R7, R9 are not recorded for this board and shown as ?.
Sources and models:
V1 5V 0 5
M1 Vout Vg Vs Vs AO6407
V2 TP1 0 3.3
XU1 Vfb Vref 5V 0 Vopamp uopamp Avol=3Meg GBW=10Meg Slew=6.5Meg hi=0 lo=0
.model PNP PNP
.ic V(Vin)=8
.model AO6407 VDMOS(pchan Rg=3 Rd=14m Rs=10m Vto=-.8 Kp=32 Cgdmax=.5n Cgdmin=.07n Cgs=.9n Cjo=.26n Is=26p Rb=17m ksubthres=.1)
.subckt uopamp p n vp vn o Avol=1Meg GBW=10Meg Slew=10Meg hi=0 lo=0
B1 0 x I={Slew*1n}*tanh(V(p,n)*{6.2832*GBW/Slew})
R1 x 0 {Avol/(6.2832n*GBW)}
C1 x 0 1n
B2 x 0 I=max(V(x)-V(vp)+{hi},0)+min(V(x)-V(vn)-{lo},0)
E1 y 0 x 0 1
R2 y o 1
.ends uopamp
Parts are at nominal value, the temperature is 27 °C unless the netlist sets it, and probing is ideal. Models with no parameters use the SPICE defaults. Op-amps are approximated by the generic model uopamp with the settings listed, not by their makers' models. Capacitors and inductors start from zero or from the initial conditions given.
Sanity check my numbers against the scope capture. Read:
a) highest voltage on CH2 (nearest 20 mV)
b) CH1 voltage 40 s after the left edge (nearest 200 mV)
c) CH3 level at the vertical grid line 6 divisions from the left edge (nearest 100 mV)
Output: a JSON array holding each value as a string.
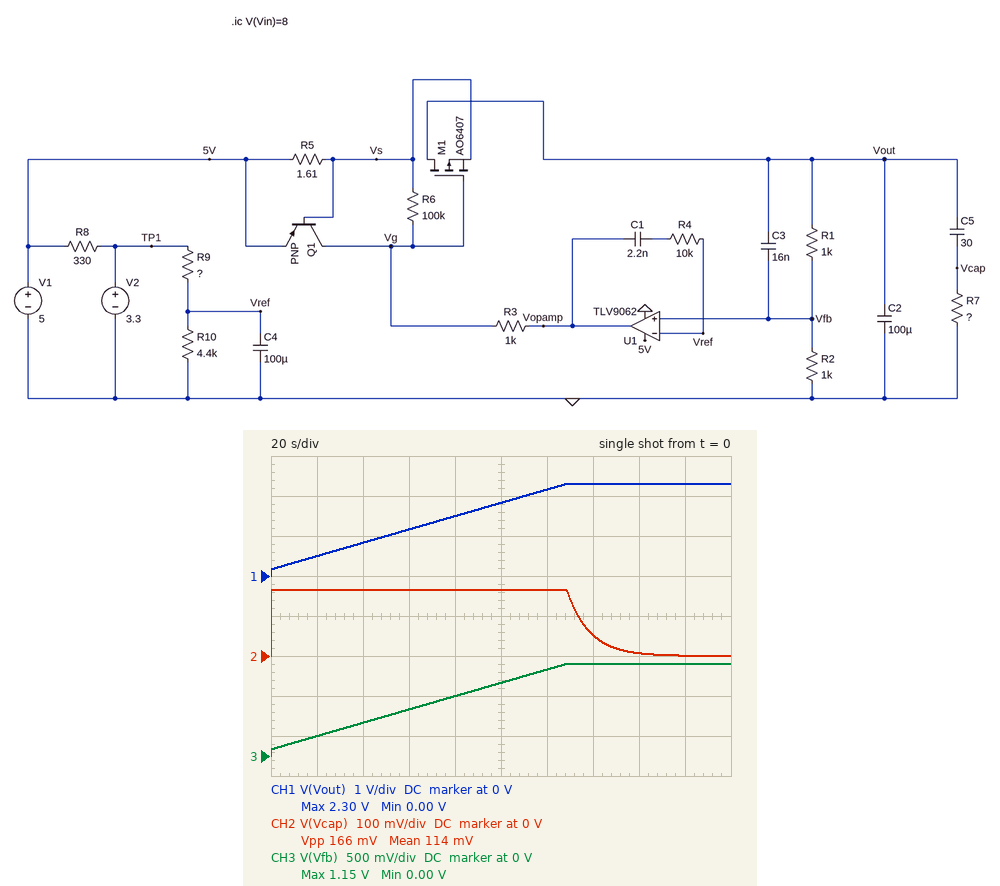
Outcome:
["160 mV", "800 mV", "1.1 V"]
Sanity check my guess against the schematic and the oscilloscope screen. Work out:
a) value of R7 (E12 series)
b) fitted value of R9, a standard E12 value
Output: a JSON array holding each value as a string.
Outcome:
["0.33 Ω", "8.2 kΩ"]
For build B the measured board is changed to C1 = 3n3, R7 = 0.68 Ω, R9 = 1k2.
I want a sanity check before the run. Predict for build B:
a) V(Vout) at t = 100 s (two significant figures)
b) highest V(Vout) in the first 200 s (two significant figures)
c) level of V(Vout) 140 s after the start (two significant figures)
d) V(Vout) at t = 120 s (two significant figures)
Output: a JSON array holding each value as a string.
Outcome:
["2.0 V", "3.7 V", "2.7 V", "2.3 V"]
